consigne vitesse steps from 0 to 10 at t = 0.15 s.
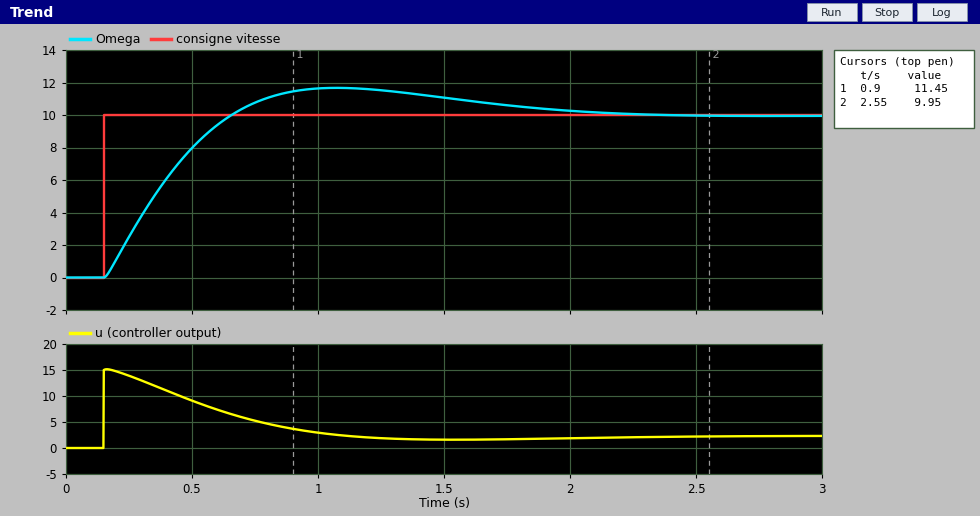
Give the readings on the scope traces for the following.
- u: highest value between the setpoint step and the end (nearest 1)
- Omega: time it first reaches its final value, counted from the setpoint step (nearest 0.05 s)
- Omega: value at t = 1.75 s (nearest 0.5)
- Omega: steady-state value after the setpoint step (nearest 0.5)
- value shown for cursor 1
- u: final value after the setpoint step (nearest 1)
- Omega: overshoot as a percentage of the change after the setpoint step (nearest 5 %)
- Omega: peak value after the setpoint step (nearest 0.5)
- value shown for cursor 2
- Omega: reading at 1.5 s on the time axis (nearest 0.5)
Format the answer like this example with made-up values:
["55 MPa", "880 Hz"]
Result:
["15", "0.50 s", "10.5", "10.0", "11.45", "2", "15 %", "11.5", "9.95", "11.0"]
